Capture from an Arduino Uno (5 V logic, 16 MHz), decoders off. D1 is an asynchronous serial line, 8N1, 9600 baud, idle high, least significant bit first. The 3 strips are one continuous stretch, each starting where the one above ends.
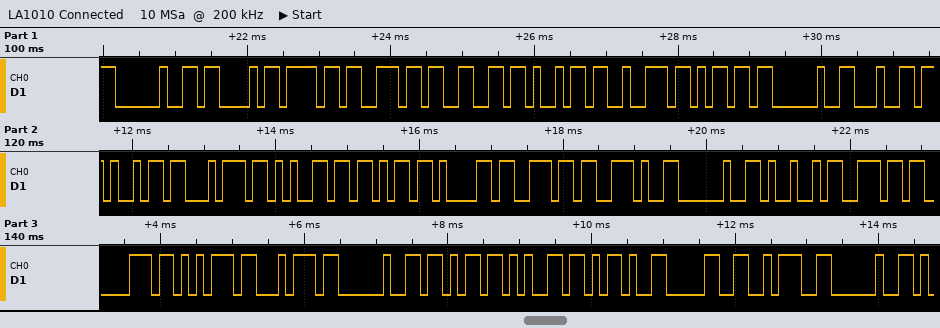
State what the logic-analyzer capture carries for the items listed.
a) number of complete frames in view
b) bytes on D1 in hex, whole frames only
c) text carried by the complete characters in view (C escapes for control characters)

30
20 43 6F 6E 66 69 72 6D 20 64 69 74 65 6B 61 6E 2E 20 49 6E 70 75 74 20 6B 65 2D 30 3A 20
" Confirm ditekan. Input ke-0: "
